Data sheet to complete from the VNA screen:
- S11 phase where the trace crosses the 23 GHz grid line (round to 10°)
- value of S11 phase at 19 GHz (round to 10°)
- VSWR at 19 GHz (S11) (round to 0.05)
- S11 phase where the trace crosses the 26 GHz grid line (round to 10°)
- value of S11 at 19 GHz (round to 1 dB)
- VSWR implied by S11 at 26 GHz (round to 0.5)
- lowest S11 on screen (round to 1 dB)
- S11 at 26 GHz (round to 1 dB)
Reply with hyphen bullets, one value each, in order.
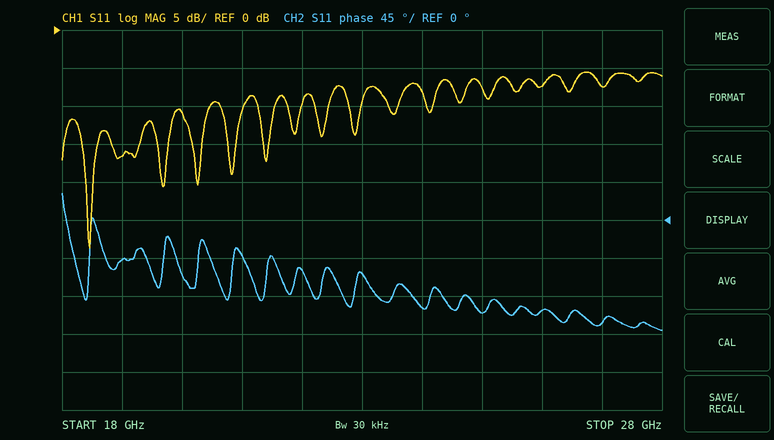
- -60°
- -50°
- 1.35
- -110°
- -17 dB
- 2.5
- -29 dB
- -7 dB
